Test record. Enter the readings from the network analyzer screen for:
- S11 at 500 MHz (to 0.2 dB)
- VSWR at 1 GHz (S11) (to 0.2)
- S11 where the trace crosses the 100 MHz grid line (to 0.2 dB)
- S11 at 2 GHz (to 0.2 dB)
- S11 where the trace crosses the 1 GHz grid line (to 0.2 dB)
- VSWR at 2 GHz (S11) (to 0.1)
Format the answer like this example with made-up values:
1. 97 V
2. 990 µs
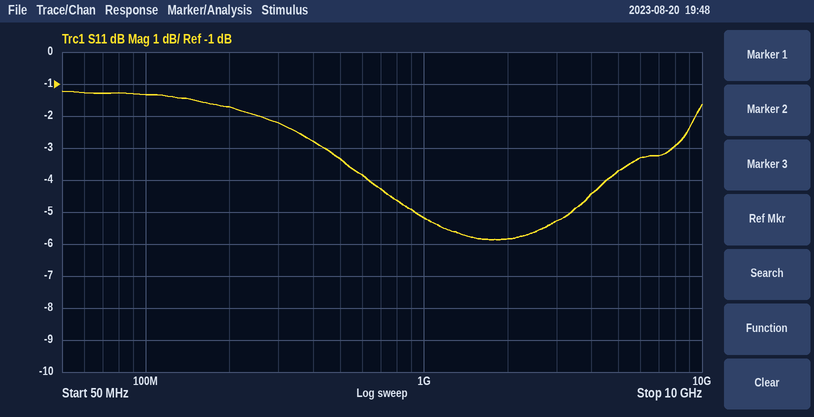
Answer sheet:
1. -3.4 dB
2. 3.4
3. -1.4 dB
4. -5.8 dB
5. -5.2 dB
6. 3.1
